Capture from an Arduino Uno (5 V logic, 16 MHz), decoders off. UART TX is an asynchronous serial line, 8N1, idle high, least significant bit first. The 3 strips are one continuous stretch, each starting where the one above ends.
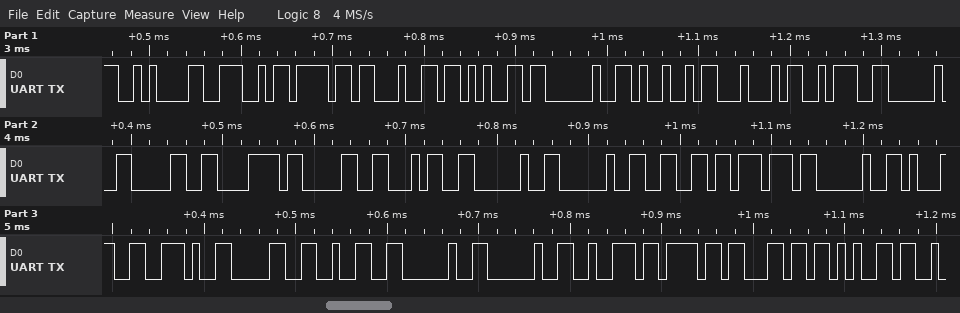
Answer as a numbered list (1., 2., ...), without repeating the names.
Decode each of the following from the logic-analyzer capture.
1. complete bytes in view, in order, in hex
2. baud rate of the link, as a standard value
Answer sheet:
1. 0A 4E 6F 64 65 20 49 44 3A 20 30 78 30 34 20 20 66 77 20 31 2E 30 32 20 20 72 6F 6C 65
2. 115200 baud
